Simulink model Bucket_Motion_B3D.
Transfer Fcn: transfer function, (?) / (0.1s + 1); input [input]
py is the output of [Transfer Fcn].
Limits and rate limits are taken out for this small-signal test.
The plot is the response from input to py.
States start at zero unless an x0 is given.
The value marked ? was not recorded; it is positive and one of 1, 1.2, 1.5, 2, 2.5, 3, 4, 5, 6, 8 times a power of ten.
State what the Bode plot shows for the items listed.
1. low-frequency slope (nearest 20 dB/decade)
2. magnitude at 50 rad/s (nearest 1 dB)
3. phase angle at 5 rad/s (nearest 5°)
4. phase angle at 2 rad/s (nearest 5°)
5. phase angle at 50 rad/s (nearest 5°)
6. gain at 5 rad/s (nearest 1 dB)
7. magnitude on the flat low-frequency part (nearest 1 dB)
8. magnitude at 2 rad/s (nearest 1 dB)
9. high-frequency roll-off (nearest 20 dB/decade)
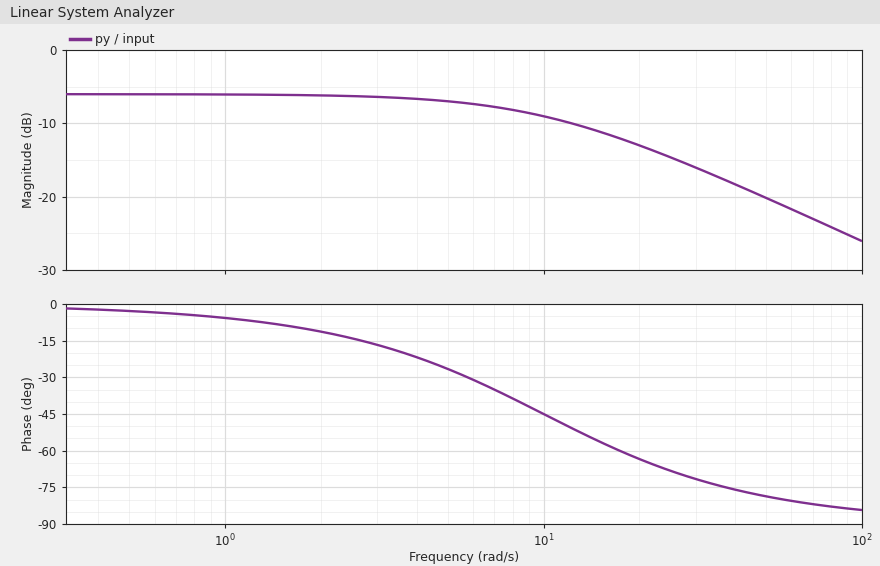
0 dB/decade
-20 dB
-25°
-10°
-80°
-7 dB
-6 dB
-6 dB
-20 dB/decade
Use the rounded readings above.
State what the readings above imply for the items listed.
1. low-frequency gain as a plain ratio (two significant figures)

0.50
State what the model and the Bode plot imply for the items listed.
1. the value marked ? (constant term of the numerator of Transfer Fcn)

0.5
